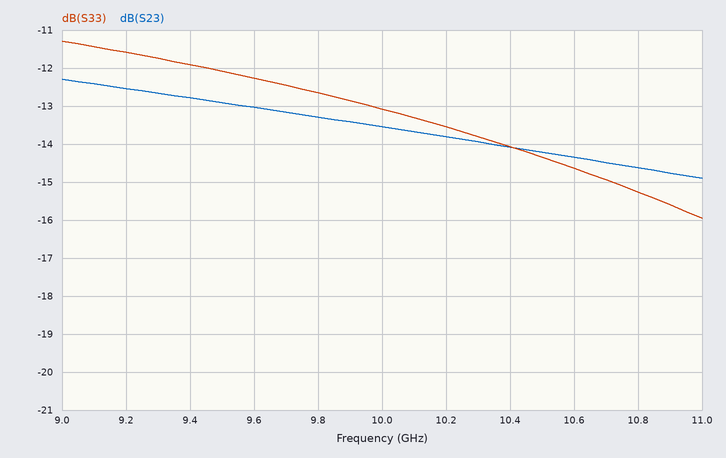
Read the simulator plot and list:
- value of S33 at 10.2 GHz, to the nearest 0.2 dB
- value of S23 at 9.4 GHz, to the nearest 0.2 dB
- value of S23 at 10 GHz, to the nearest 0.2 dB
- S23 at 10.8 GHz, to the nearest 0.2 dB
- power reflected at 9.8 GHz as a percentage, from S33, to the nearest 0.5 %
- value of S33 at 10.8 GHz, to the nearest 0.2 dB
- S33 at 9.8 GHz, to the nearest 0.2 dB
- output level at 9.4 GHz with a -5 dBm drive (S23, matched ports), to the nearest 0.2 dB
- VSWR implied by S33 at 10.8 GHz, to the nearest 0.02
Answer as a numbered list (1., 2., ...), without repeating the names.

1. -13.6 dB
2. -12.8 dB
3. -13.6 dB
4. -14.6 dB
5. 5.5 %
6. -15.2 dB
7. -12.6 dB
8. -17.8 dBm
9. 1.42
